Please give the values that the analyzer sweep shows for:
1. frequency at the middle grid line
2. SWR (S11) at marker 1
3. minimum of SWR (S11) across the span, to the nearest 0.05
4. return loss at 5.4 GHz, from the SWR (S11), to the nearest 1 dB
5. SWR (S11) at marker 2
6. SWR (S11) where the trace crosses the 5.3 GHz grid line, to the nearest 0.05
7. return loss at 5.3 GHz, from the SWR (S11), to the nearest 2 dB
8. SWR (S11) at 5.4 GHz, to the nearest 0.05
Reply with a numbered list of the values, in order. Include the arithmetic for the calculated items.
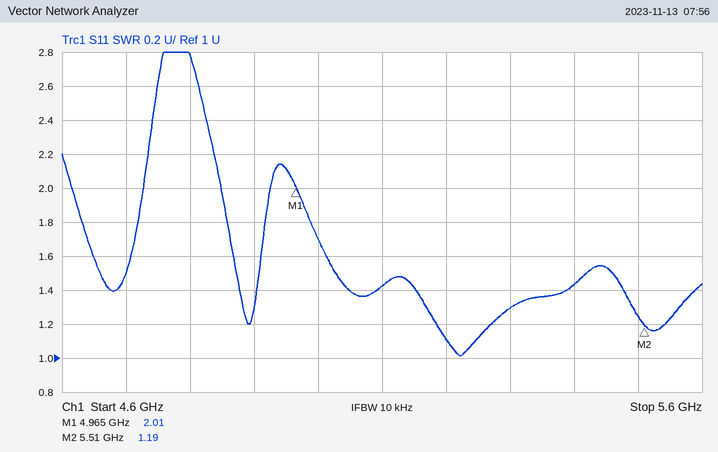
1. 5.1 GHz
2. 2.01
3. 1.00
4. −20 log10((1.45 − 1)/(1.45 + 1)) ≈ 15 dB
5. 1.19
6. 1.30
7. −20 log10((1.3 − 1)/(1.3 + 1)) ≈ 18 dB
8. 1.45
